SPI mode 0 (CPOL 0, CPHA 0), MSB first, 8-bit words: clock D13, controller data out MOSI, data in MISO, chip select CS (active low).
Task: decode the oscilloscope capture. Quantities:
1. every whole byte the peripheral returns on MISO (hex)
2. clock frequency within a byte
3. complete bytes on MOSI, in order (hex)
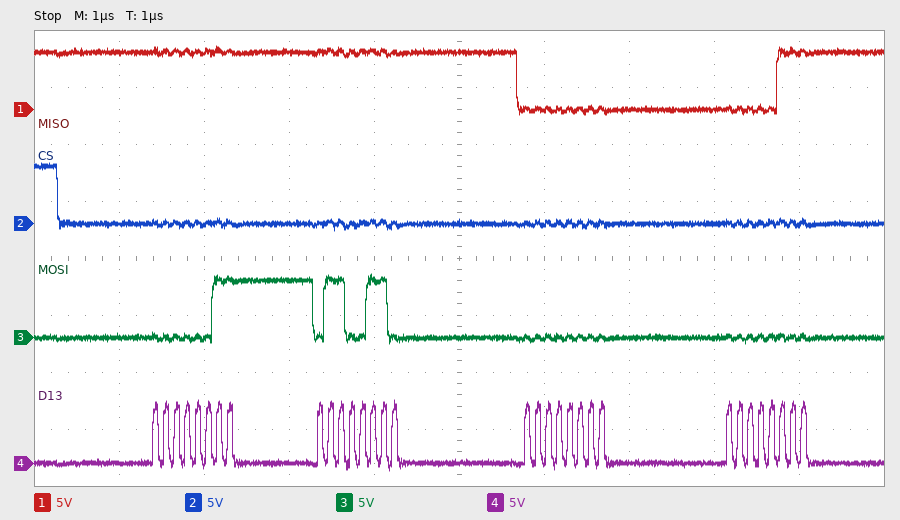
FF FF 00 07
8 MHz
03 66 00 00
